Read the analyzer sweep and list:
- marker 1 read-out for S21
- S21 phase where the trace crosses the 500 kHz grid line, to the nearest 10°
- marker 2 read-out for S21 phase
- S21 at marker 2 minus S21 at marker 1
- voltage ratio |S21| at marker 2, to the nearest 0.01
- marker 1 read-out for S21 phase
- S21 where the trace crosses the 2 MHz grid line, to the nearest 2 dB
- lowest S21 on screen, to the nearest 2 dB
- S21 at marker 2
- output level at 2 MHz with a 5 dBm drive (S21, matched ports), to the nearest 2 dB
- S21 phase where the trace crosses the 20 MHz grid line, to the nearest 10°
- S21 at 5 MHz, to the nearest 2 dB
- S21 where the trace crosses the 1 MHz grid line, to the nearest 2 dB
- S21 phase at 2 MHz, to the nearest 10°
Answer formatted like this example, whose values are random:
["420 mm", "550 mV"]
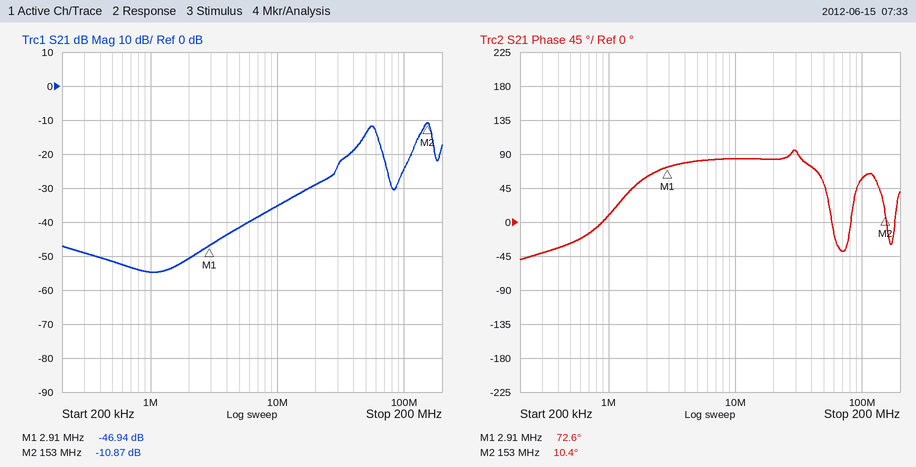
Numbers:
["-46.94 dB", "-30°", "10.4°", "36.07 dB", "0.29", "72.6°", "-50 dB", "-54 dB", "-10.87 dB", "-46 dBm", "80°", "-42 dB", "-54 dB", "60°"]
